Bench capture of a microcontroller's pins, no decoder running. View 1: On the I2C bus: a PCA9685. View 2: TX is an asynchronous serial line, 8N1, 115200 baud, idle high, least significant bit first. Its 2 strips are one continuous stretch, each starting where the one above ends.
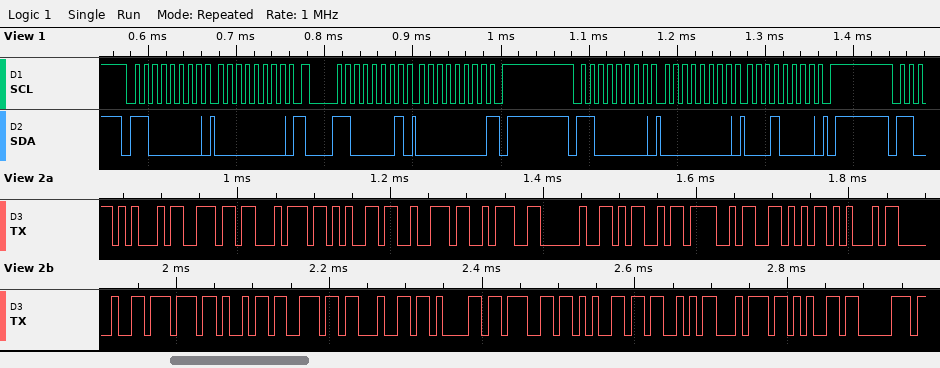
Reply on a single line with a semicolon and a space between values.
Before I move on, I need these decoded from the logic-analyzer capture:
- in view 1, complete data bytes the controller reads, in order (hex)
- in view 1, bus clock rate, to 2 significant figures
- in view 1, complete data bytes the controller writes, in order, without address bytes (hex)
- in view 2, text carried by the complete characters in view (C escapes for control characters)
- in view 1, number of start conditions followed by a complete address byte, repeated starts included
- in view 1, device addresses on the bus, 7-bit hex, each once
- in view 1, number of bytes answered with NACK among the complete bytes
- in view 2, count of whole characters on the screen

00; 100 kHz; 00 00 10; "Enter: MOVE windageStep"; 3; 0x60; 1; 23
